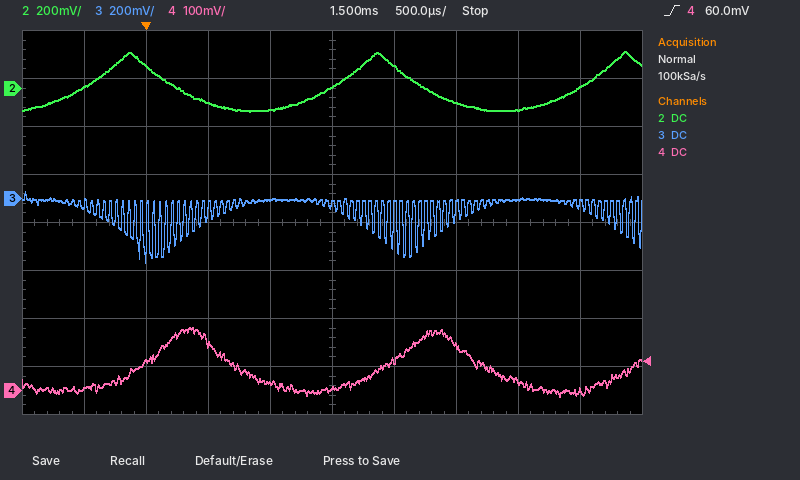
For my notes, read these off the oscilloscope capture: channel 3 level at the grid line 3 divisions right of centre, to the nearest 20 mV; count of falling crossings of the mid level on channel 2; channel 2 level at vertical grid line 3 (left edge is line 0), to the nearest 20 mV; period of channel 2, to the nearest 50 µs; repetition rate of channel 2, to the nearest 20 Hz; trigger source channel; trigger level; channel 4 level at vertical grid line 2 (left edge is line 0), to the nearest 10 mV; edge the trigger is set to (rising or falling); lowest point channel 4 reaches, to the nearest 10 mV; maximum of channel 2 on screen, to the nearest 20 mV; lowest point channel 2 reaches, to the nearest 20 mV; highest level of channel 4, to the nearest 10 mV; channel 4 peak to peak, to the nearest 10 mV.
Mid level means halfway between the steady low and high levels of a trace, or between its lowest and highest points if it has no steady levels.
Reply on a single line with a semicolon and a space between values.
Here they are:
0 mV; 2; -60 mV; 2.00 ms; 500 Hz; channel 4; 60.0 mV; 60 mV; rising; -10 mV; 160 mV; -100 mV; 130 mV; 140 mV
